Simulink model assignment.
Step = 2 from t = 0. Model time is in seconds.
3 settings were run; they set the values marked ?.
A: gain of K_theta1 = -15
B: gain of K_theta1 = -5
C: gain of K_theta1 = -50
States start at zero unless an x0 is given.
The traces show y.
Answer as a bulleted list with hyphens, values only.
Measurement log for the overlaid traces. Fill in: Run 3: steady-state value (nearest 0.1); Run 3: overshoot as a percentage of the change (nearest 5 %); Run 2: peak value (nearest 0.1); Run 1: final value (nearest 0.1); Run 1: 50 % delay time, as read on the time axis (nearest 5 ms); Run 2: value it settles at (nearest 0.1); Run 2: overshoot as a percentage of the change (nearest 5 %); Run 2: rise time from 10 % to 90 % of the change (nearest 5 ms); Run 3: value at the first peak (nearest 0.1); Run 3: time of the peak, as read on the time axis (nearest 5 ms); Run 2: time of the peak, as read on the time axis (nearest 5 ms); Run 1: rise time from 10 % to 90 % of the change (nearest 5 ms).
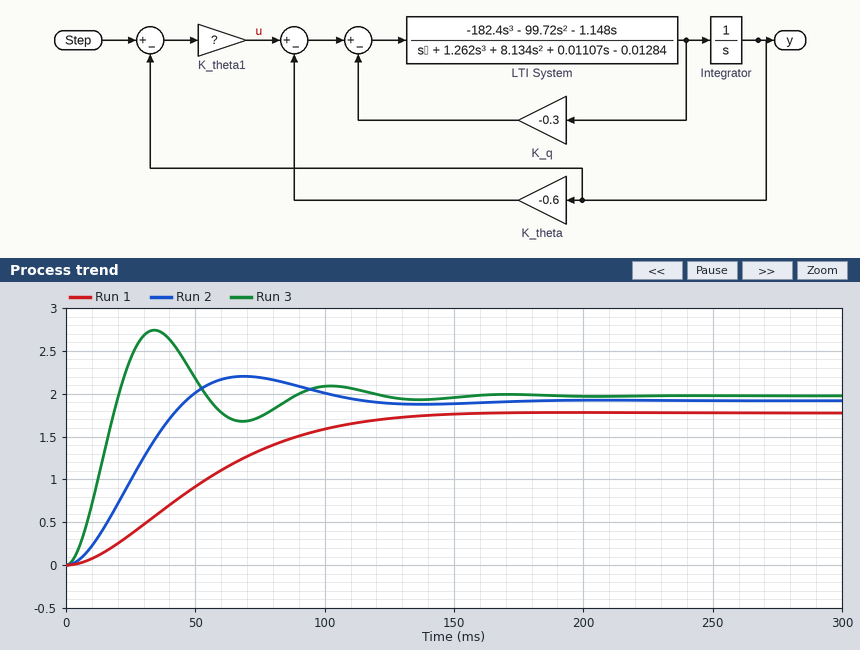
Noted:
- 2.0
- 40 %
- 2.2
- 1.8
- 50 ms
- 1.9
- 15 %
- 30 ms
- 2.7
- 35 ms
- 70 ms
- 85 ms
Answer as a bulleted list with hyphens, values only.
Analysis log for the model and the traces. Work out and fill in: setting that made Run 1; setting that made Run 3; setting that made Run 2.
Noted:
- B
- C
- A
